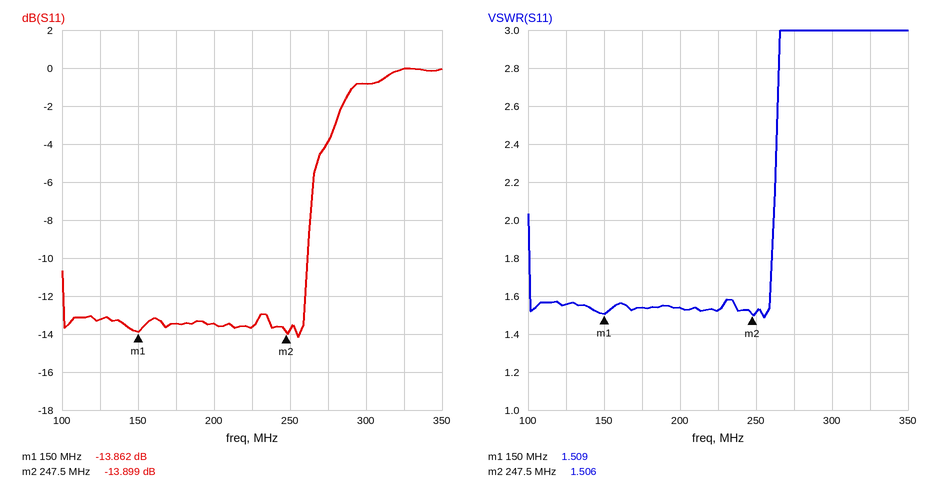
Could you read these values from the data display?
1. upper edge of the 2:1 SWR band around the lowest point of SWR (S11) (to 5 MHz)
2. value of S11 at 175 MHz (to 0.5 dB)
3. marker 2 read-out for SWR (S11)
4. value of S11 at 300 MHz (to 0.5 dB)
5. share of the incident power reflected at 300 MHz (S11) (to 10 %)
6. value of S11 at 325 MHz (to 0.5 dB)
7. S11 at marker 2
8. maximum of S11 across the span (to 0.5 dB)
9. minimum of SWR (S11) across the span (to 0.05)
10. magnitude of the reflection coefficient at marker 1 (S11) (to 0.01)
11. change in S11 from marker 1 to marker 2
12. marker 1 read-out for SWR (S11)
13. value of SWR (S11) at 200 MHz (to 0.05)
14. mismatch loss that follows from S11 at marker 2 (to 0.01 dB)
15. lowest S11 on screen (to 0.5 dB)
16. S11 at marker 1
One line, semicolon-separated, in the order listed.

260 MHz; -13.5 dB; 1.506; -1.0 dB; 80 %; 0.0 dB; -13.899 dB; 0.0 dB; 1.50; 0.20; -0.037 dB; 1.509; 1.55; 0.18 dB; -14.0 dB; -13.862 dB
